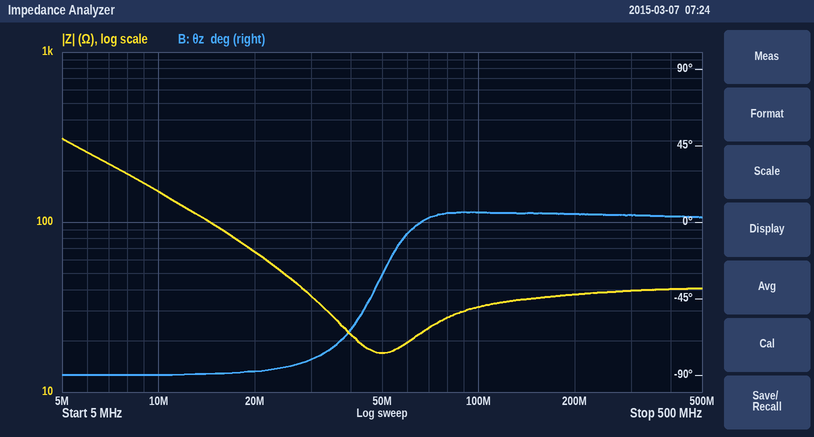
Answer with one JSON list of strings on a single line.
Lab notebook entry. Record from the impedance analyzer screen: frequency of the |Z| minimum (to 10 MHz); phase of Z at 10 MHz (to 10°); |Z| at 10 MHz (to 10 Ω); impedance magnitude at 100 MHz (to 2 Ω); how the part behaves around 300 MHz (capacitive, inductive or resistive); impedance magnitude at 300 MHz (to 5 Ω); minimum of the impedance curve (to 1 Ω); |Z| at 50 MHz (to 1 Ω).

["50 MHz", "-90°", "150 Ω", "32 Ω", "resistive", "40 Ω", "17 Ω", "17 Ω"]
